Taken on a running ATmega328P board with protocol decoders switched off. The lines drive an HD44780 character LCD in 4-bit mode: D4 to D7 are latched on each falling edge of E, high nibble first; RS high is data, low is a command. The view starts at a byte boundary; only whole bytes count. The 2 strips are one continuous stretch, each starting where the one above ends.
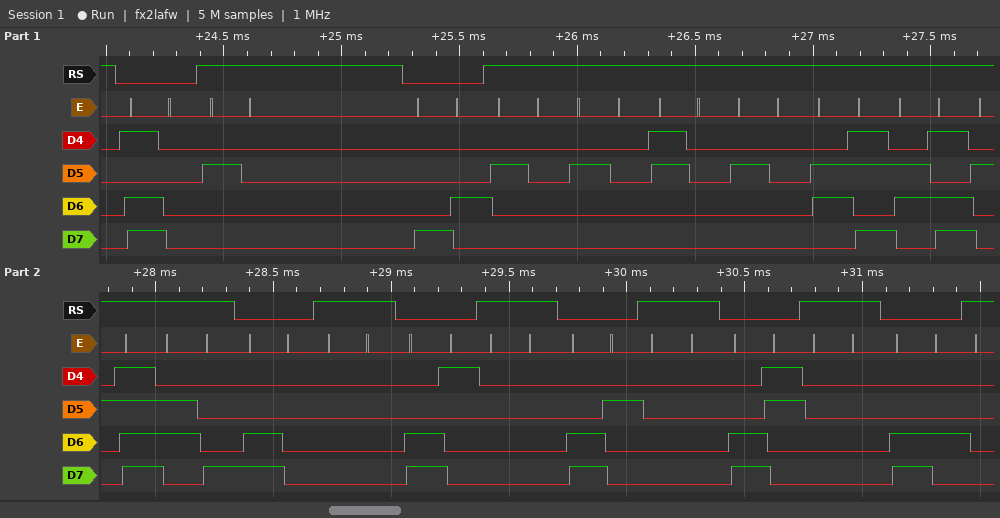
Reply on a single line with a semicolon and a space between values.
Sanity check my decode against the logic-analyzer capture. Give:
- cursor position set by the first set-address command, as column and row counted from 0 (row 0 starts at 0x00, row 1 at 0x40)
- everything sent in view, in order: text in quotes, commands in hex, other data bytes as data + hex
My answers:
column 16, row 1; 0xD0 " " 0x84 "  0 km/h" 0xC0 data 00 0xC1 data 00 0xC2 data 00 0xC3 data 00 0xC4
